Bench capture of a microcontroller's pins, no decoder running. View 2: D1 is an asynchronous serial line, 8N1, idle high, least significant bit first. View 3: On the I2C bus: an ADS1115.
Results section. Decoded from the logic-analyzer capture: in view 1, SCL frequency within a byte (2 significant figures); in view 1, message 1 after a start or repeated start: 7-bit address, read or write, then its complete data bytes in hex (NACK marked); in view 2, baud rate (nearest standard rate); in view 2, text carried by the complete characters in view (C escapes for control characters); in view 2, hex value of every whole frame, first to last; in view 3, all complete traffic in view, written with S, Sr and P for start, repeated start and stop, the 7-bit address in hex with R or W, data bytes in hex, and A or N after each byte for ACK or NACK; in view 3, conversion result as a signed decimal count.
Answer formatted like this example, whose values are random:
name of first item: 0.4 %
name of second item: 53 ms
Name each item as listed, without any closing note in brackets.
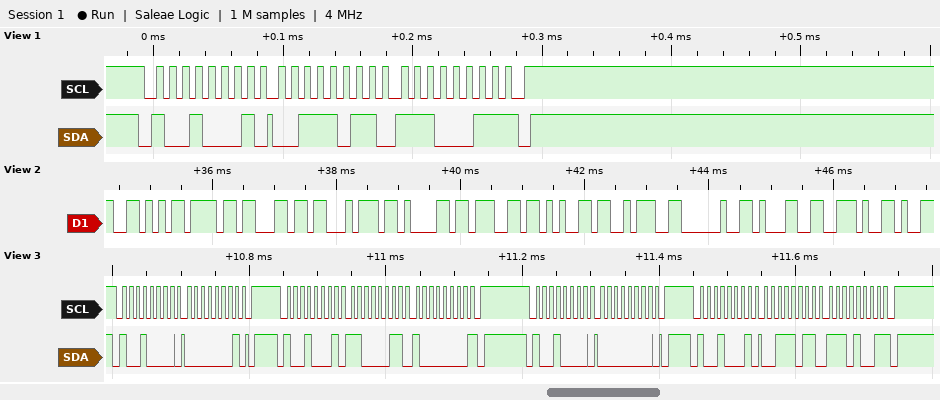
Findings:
in view 1, SCL frequency within a byte: 100 kHz
in view 1, message 1 after a start or repeated start: 7-bit address, read or write, then its complete data bytes in hex: 0x48 read: 3B E3 NACK
in view 2, baud rate: 9600 baud
in view 2, text carried by the complete characters in view: "Voltage: 1."
in view 2, hex value of every whole frame, first to last: 56 6F 6C 74 61 67 65 3A 20 31 2E
in view 3, all complete traffic in view, written with S, Sr and P for start, repeated start and stop, the 7-bit address in hex with R or W, data bytes in hex, and A or N after each byte for ACK or NACK: S 48W A 01 A P S 48R A C3 A 80 N P S 48W A 00 A P S 48R A 3B A E9 N P
in view 3, conversion result as a signed decimal count: 15337
